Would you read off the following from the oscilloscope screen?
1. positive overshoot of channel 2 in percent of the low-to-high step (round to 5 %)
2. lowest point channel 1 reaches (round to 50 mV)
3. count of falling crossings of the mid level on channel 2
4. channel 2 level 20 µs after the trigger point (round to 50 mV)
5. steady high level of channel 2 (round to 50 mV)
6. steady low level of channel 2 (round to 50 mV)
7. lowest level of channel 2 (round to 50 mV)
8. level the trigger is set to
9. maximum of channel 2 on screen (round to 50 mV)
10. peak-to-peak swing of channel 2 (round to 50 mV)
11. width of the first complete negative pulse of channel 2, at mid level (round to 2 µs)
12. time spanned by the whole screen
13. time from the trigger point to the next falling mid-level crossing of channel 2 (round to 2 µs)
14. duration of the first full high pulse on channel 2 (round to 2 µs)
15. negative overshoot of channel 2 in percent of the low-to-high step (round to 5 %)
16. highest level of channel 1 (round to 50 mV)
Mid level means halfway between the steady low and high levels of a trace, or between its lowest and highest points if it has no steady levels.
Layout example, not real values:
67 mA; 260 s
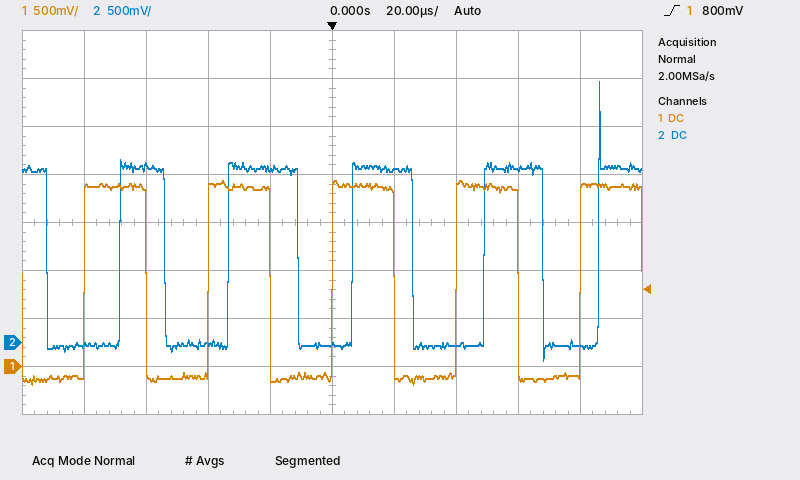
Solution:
50 %; -200 mV; 5; 1.80 V; 1.80 V; -50 mV; -200 mV; 800 mV; 2.70 V; 2.90 V; 24 µs; 200 µs; 26 µs; 14 µs; 10 %; 1.95 V
